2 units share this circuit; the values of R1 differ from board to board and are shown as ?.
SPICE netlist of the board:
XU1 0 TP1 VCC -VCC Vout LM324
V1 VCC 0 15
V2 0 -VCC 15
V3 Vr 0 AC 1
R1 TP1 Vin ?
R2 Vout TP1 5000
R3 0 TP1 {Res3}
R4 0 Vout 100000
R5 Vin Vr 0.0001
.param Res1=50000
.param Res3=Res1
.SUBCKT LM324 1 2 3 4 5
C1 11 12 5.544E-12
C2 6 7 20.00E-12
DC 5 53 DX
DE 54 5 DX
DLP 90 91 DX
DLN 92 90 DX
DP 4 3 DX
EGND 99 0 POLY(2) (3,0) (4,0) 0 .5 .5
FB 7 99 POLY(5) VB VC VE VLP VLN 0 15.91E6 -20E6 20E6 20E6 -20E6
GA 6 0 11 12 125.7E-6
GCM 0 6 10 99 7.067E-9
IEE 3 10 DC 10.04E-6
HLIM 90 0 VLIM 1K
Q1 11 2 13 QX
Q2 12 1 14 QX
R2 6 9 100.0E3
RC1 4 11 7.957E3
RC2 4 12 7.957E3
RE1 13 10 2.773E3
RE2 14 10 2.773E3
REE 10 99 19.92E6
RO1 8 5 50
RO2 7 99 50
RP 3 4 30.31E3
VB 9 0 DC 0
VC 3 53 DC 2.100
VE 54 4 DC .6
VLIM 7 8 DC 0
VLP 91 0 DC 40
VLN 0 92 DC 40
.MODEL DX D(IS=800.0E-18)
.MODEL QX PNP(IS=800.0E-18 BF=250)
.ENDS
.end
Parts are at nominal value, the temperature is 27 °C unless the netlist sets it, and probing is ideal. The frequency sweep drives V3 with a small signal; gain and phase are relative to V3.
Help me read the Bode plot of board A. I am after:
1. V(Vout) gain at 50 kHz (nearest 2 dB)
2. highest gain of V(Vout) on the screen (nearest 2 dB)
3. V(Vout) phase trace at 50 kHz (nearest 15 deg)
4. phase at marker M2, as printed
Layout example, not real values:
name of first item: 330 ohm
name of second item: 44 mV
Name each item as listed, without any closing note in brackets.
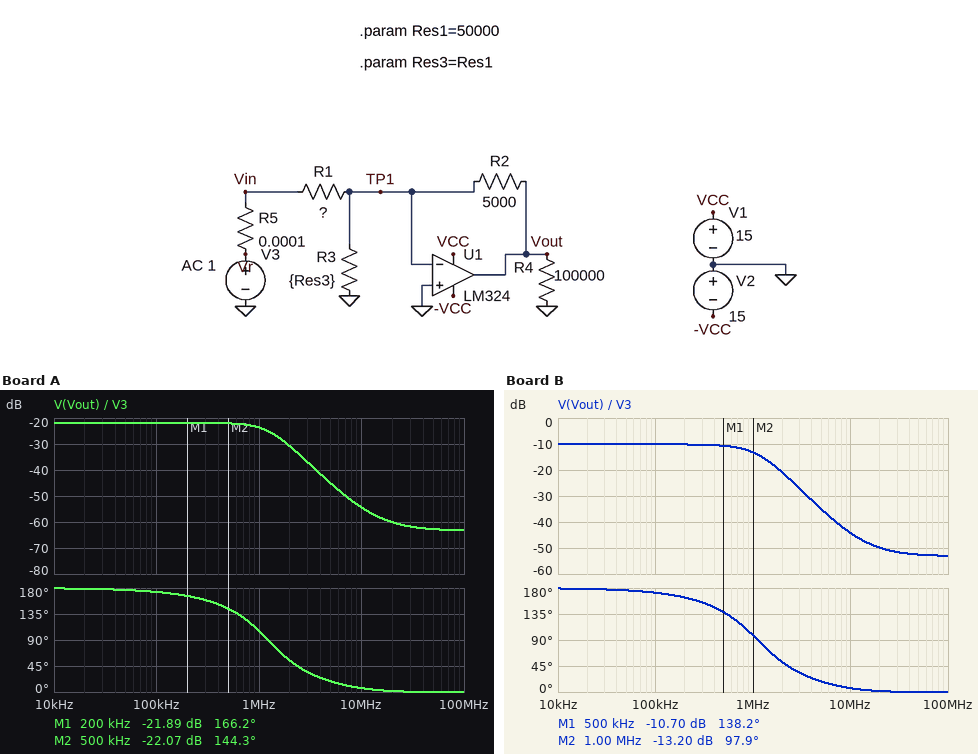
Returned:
V(Vout) gain at 50 kHz: -22 dB
highest gain of V(Vout) on the screen: -22 dB
V(Vout) phase trace at 50 kHz: 180 deg
phase at marker M2, as printed: 144.3 deg
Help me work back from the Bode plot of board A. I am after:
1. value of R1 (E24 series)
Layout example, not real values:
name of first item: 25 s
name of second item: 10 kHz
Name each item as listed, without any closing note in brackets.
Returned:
value of R1: 62 kΩ
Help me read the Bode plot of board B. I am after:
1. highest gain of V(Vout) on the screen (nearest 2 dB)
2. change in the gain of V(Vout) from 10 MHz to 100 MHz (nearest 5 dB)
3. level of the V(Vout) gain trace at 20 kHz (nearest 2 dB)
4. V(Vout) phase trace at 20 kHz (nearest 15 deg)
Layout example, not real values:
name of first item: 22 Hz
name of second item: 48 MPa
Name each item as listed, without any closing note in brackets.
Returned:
highest gain of V(Vout) on the screen: -10 dB
change in the gain of V(Vout) from 10 MHz to 100 MHz: -10 dB
level of the V(Vout) gain trace at 20 kHz: -10 dB
V(Vout) phase trace at 20 kHz: 180 deg
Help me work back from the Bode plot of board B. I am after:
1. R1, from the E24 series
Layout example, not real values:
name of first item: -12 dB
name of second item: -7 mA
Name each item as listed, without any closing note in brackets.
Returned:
R1, from the E24 series: 16 kΩ
